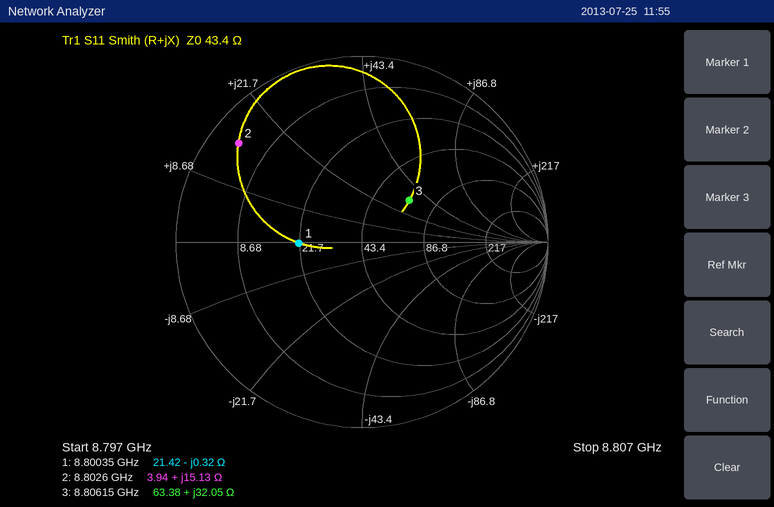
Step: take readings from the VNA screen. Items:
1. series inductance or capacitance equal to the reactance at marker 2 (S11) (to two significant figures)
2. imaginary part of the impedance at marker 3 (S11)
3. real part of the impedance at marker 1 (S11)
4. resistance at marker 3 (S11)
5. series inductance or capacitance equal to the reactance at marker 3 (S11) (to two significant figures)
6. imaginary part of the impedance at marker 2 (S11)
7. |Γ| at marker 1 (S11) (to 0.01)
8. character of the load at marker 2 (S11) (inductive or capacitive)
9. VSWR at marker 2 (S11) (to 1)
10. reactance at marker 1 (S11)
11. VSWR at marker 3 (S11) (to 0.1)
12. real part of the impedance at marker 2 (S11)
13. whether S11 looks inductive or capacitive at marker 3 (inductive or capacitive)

270 pH
+32.05 Ω
21.42 Ω
63.38 Ω
580 pH
+15.13 Ω
0.34
inductive
12
-0.32 Ω
2.0
3.94 Ω
inductive
